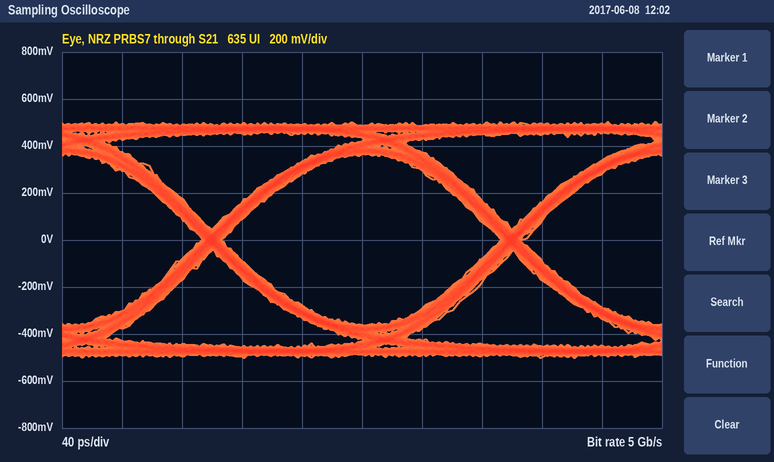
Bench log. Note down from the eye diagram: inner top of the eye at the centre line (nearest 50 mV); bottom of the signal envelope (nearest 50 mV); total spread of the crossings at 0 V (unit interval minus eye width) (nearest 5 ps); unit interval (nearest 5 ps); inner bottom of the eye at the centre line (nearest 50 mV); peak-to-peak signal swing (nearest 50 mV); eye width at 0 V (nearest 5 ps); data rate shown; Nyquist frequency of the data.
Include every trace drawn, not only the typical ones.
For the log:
350 mV
-500 mV
15 ps
200 ps
-350 mV
1.00 V
185 ps
5 Gb/s
2.5 GHz
